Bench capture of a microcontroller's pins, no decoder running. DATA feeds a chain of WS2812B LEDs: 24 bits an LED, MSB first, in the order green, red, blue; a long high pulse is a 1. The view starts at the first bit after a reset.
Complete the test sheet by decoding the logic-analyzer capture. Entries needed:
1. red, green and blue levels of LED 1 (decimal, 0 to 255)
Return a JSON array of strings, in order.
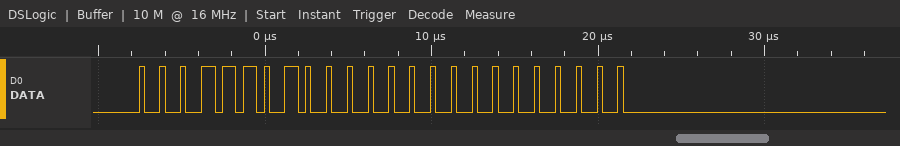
["0, 29, 0"]
